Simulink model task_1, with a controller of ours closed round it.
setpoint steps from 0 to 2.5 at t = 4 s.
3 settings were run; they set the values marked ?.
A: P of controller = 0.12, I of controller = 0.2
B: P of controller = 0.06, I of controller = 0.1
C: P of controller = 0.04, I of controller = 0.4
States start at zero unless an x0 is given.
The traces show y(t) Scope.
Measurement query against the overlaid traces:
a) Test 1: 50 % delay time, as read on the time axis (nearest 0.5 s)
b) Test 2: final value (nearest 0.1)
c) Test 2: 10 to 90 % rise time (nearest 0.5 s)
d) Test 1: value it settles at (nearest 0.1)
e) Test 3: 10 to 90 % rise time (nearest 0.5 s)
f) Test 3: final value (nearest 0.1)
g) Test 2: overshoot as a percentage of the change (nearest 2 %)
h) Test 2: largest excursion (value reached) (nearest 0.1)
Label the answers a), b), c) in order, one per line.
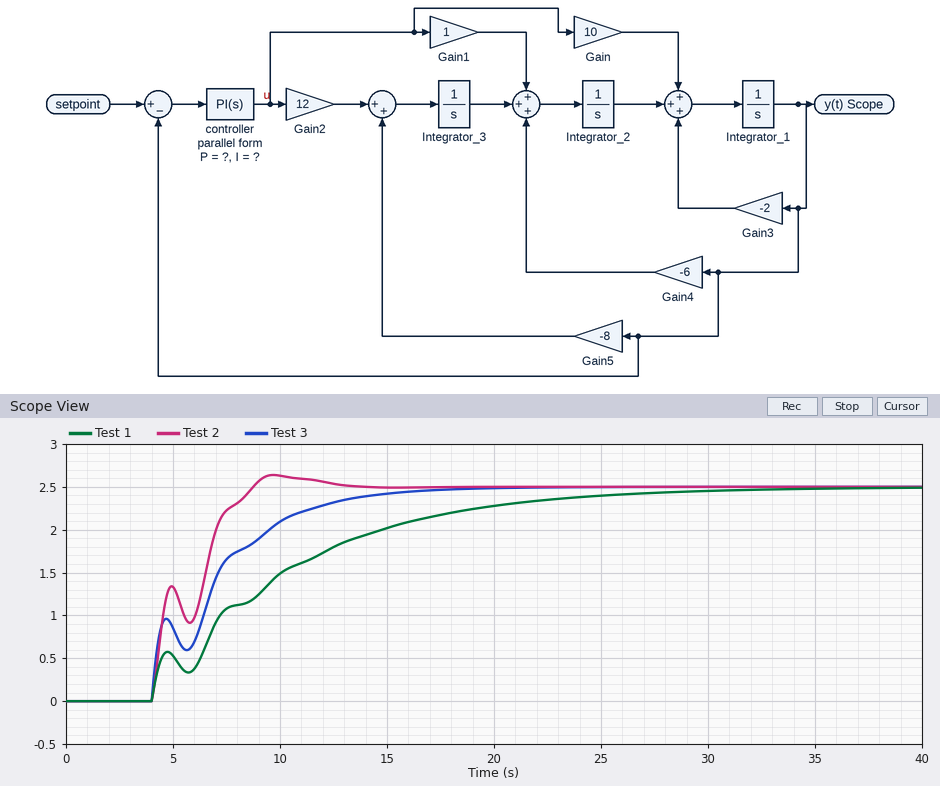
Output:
a) 9.0 s
b) 2.5
c) 3.5 s
d) 2.5
e) 7.5 s
f) 2.5
g) 6 %
h) 2.6
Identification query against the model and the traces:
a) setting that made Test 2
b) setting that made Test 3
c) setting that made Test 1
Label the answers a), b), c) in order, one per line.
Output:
a) C
b) A
c) B
